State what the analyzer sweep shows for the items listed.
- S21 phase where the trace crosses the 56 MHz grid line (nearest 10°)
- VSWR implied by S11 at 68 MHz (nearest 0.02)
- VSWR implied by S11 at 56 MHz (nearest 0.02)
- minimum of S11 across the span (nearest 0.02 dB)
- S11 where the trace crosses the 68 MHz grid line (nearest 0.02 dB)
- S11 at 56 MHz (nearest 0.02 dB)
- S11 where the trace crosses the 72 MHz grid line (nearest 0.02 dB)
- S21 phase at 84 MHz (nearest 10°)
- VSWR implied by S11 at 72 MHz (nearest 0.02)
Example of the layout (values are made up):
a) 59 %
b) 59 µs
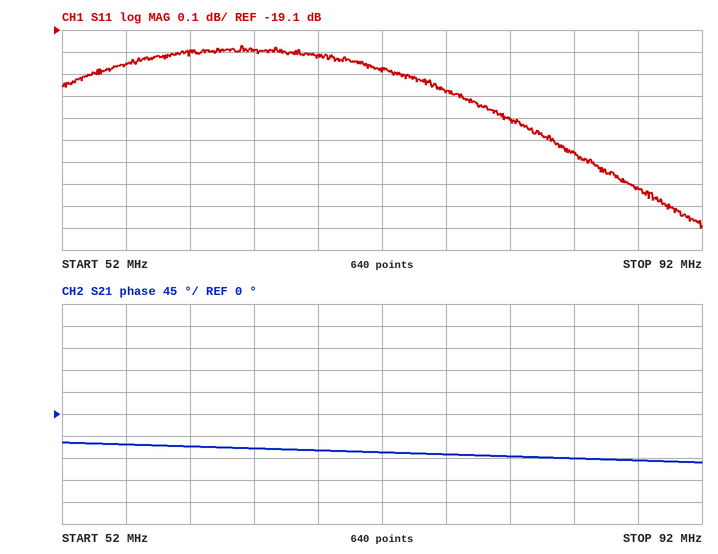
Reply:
a) -60°
b) 1.24
c) 1.24
d) -20.00 dB
e) -19.22 dB
f) -19.26 dB
g) -19.28 dB
h) -90°
i) 1.24
